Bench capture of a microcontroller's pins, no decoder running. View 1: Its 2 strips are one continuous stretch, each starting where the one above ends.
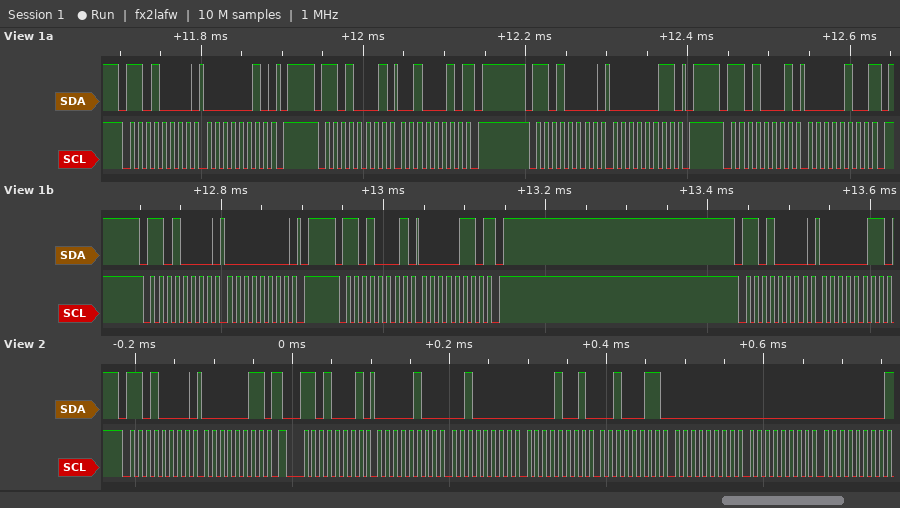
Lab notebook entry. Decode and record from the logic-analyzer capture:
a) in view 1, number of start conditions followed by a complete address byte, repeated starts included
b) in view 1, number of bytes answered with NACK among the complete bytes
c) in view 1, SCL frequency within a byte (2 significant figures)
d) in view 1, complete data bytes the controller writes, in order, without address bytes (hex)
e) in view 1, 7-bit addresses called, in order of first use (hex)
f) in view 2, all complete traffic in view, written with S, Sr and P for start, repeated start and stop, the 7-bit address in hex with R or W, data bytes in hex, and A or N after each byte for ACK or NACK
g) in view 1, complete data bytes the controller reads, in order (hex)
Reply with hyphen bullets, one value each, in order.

- 7
- 3
- 100 kHz
- 02 03 00 03
- 0x68
- S 68W A 03 A Sr 68R A 04 A 20 A 09 A 23 A 00 A 00 A 00 N
- 22 04 06
